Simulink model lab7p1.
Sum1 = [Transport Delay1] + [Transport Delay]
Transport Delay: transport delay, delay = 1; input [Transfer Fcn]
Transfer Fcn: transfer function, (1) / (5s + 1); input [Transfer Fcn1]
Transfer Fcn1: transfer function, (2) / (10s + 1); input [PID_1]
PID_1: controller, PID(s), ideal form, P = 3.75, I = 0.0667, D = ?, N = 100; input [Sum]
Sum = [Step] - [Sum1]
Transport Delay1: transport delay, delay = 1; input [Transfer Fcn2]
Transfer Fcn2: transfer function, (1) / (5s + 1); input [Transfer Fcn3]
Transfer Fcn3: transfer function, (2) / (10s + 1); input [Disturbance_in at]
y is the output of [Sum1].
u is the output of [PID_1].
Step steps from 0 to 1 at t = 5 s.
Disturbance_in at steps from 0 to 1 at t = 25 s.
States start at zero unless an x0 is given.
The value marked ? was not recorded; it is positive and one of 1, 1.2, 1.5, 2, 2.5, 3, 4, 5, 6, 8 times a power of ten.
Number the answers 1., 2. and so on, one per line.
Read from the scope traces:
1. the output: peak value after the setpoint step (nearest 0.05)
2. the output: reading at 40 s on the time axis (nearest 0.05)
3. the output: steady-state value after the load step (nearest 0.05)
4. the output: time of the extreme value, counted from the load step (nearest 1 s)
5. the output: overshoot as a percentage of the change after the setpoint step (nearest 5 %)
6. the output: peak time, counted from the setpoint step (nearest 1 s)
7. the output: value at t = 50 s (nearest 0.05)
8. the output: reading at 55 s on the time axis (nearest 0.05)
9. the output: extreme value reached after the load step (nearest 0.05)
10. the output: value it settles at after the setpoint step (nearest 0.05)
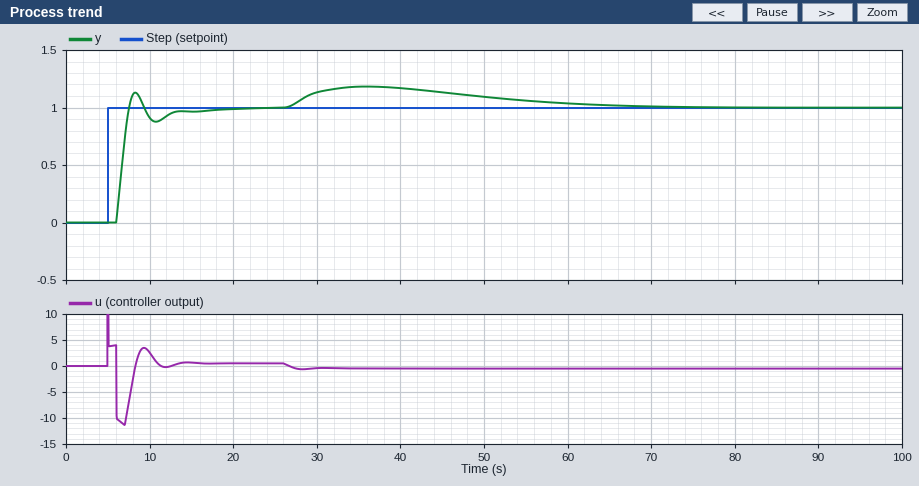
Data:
1. 1.15
2. 1.15
3. 1.00
4. 11 s
5. 15 %
6. 3 s
7. 1.10
8. 1.05
9. 1.20
10. 1.00
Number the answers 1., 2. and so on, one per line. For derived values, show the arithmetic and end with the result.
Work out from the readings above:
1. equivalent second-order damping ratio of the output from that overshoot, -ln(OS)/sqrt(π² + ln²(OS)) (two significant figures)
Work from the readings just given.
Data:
1. ln(0.15) = -1.897; 1.897 / sqrt(9.870 + 3.599) = 0.52
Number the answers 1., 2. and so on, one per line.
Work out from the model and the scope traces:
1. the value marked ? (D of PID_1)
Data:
1. 5
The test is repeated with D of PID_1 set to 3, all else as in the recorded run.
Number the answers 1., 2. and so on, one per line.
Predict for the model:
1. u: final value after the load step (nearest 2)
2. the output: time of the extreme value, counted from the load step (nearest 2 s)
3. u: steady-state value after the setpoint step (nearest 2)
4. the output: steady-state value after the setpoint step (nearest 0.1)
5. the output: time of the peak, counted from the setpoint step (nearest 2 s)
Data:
1. 0
2. 8 s
3. 0
4. 1.0
5. 6 s
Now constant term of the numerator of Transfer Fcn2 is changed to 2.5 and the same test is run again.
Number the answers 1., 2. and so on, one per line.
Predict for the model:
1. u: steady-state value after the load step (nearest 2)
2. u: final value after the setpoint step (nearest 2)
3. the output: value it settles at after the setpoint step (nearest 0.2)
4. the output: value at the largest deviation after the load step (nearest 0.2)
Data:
1. -2
2. 0
3. 1.0
4. 1.4
